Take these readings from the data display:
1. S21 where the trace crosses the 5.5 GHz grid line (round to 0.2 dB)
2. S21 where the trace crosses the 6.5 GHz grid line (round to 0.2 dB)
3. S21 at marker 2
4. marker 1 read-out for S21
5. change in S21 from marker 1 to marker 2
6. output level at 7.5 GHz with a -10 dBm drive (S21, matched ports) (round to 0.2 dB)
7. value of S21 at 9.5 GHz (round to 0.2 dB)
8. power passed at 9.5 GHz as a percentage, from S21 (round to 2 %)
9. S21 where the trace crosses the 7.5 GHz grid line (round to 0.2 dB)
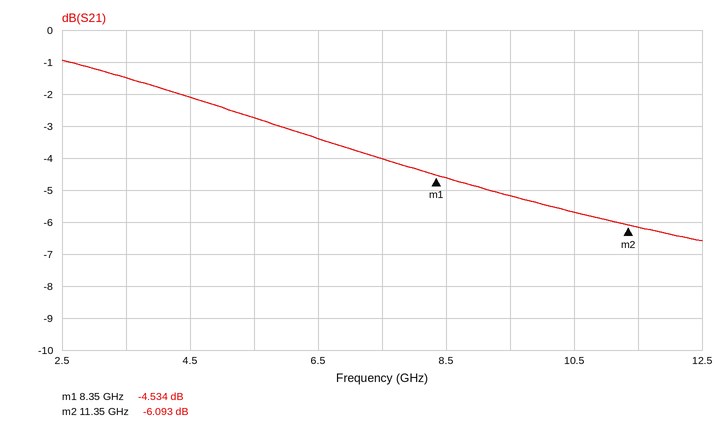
-2.8 dB
-3.4 dB
-6.093 dB
-4.534 dB
-1.559 dB
-14.0 dBm
-5.2 dB
30 %
-4.0 dB
